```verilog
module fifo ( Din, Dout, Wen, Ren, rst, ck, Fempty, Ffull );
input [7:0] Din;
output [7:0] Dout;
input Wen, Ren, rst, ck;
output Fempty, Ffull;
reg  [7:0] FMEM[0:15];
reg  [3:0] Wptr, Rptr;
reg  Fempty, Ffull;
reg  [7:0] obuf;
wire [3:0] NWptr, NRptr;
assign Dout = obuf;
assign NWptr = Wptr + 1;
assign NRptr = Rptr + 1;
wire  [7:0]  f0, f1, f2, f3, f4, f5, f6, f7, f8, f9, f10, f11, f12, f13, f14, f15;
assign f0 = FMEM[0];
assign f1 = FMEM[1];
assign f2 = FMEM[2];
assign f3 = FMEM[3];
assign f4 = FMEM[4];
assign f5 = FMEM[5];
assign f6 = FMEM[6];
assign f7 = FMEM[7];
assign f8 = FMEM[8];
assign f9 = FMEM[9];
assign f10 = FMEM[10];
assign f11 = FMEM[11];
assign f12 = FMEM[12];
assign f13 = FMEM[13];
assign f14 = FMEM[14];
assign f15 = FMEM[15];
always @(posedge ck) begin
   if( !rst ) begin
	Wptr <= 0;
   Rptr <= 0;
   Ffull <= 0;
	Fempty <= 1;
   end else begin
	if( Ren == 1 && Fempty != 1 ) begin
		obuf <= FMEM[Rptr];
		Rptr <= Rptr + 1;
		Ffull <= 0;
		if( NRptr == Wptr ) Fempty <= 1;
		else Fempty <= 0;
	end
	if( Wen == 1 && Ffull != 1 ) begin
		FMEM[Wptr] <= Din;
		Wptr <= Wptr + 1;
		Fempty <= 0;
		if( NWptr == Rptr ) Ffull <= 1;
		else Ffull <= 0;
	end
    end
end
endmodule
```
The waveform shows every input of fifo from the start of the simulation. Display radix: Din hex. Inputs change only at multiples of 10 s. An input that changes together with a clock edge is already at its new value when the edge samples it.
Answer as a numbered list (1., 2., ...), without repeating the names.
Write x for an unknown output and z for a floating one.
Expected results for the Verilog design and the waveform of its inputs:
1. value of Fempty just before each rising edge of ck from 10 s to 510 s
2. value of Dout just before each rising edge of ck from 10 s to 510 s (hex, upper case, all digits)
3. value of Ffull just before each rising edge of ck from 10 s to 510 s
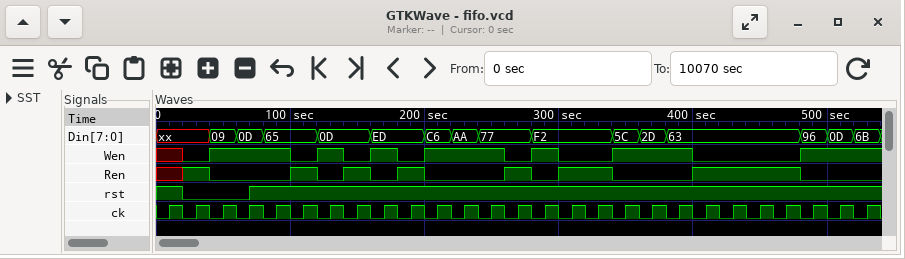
1. x x 1 1 0 0 0 0 0 0 0 0 0 0 0 0 0 0 0 0 0 0 0 0 0 0
2. x, x, x, x, x, x, 0D, 0D, 65, 65, 0D, 0D, 0D, 0D, ED, ED, C6, AA, AA, AA, AA, 77, F2, 5C, 2D, 2D
3. x x 0 0 0 0 0 0 0 0 0 0 0 0 0 0 0 0 0 0 0 0 0 0 0 0
